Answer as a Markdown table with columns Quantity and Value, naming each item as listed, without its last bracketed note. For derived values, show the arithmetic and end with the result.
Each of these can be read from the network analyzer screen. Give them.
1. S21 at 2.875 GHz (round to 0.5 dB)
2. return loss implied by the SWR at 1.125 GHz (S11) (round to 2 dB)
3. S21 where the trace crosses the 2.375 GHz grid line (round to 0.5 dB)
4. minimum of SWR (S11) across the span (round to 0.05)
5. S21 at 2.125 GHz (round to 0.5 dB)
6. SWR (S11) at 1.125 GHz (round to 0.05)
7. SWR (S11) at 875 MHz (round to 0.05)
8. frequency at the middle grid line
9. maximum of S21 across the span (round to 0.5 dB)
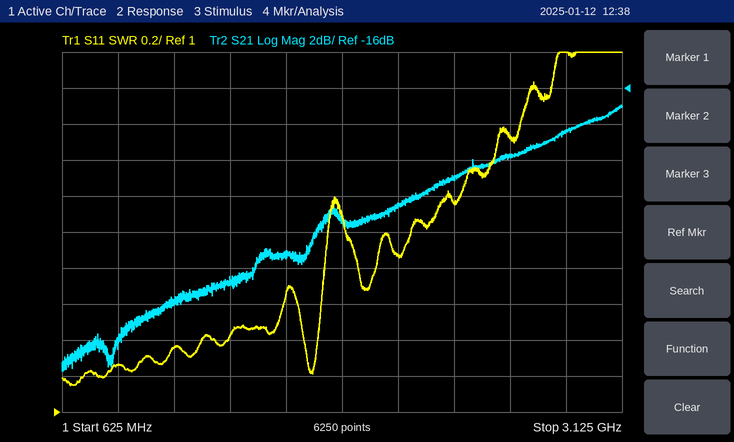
| Quantity | Value |
|---|---|
| S21 at 2.875 GHz | -18.5 dB |
| return loss implied by the SWR at 1.125 GHz (S11) | −20 log10((1.35 − 1)/(1.35 + 1)) ≈ 16 dB |
| S21 where the trace crosses the 2.375 GHz grid line | -21.0 dB |
| minimum of SWR (S11) across the span | 1.15 |
| S21 at 2.125 GHz | -22.5 dB |
| SWR (S11) at 1.125 GHz | 1.35 |
| SWR (S11) at 875 MHz | 1.25 |
| frequency at the middle grid line | 1.875 GHz |
| maximum of S21 across the span | -17.0 dB |
